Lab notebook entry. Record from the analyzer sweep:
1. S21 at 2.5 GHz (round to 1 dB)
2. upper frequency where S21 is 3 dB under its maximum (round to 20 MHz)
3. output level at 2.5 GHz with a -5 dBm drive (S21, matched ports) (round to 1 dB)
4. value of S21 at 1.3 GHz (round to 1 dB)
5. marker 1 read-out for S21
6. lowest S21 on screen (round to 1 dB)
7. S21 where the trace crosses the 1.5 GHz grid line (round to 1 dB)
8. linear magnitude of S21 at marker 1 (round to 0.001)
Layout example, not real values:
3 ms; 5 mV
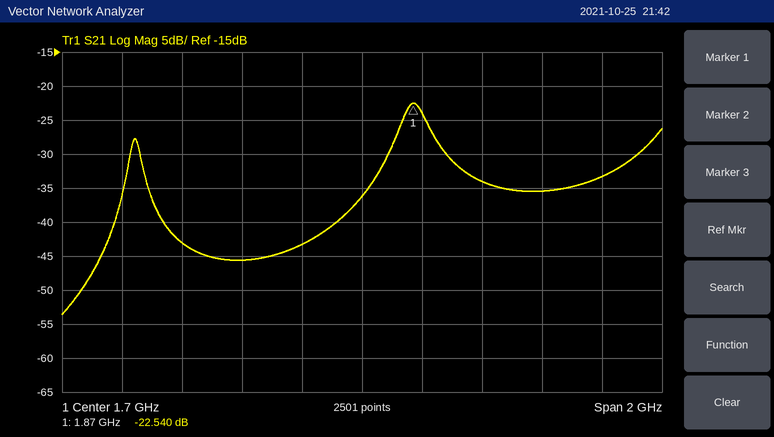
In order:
-33 dB; 1.92 GHz; -38 dBm; -46 dB; -22.540 dB; -54 dB; -43 dB; 0.075
